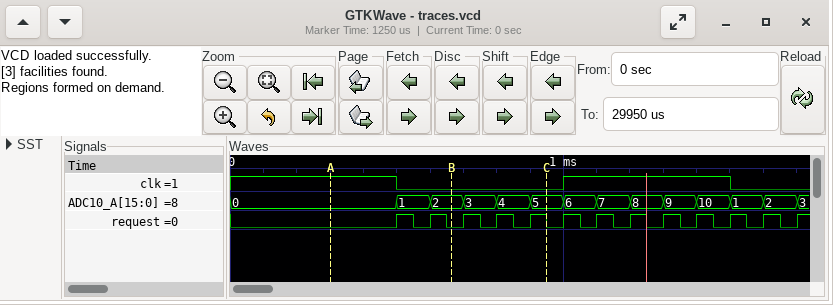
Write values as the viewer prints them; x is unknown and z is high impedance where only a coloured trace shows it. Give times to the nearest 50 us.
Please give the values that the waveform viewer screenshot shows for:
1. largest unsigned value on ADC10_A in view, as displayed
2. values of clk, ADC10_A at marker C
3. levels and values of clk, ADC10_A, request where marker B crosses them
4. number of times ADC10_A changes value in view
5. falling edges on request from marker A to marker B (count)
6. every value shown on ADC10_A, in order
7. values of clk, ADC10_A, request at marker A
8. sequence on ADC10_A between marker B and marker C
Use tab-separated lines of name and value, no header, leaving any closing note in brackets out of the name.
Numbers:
largest unsigned value on ADC10_A in view, as displayed	10
values of clk, ADC10_A at marker C	clk=0, ADC10_A=5
levels and values of clk, ADC10_A, request where marker B crosses them	clk=0, ADC10_A=2, request=0
number of times ADC10_A changes value in view	13
falling edges on request from marker A to marker B	2
every value shown on ADC10_A, in order	0, 1, 2, 3, 4, 5, 6, 7, 8, 9, 10, 1, 2, 3
values of clk, ADC10_A, request at marker A	clk=1, ADC10_A=0, request=0
sequence on ADC10_A between marker B and marker C	2, 3, 4, 5
